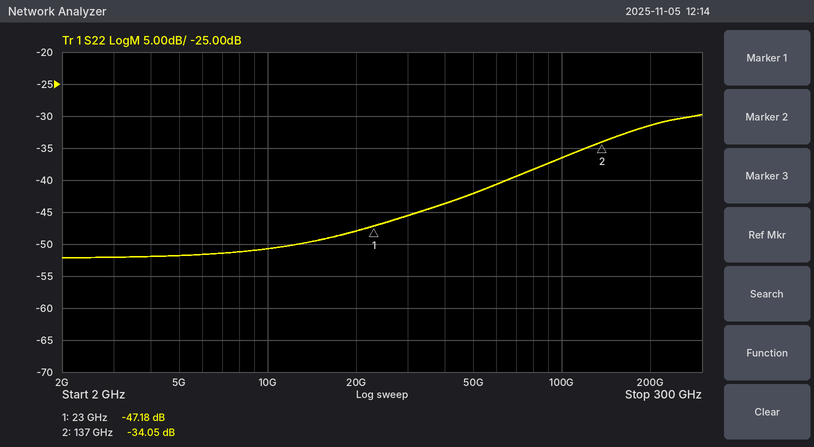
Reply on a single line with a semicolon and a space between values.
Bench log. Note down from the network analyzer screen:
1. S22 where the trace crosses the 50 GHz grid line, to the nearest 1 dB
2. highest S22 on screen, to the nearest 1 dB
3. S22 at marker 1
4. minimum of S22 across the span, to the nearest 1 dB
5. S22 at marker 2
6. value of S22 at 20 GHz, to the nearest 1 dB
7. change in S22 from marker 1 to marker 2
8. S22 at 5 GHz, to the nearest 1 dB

-42 dB; -30 dB; -47.18 dB; -52 dB; -34.05 dB; -48 dB; 13.13 dB; -52 dB
